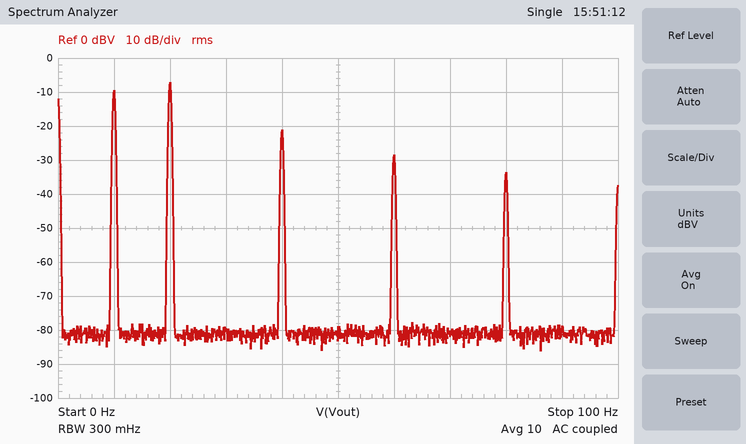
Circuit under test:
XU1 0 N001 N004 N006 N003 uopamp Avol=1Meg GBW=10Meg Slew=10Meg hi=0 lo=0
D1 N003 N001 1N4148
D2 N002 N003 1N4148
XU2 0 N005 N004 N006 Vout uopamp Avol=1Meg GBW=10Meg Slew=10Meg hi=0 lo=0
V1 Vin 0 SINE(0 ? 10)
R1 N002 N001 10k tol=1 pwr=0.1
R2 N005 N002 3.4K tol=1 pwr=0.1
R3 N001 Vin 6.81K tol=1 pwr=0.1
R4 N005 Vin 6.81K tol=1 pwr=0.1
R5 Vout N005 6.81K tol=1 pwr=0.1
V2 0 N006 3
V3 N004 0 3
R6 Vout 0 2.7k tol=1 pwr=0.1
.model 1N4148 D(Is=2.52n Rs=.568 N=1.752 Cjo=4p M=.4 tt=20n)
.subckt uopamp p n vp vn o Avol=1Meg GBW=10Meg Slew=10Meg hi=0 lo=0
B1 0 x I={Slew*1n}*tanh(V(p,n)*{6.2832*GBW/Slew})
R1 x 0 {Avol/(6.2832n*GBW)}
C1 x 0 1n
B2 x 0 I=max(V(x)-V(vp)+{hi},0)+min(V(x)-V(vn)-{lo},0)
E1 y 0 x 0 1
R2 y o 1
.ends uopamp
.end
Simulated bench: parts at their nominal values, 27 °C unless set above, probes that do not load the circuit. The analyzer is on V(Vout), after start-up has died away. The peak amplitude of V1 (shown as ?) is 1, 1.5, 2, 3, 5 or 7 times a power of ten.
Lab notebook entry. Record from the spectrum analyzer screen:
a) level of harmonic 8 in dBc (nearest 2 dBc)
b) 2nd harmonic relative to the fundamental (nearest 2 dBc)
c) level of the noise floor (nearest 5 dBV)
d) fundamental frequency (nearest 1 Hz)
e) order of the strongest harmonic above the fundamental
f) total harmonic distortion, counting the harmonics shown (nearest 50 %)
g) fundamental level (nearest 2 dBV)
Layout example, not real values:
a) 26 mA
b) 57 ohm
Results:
a) -24 dBc
b) 2 dBc
c) -80 dBV
d) 10 Hz
e) 2
f) 150 %
g) -10 dBV
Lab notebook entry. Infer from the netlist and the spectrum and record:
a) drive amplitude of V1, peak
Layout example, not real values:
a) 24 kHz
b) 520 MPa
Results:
a) 1 V
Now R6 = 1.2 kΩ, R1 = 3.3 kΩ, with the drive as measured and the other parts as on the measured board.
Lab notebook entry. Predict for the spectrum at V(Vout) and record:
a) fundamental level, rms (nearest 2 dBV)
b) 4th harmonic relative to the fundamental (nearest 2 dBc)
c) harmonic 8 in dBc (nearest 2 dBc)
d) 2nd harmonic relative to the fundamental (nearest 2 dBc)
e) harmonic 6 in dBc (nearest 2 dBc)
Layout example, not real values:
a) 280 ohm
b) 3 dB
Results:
a) -8 dBV
b) -22 dBc
c) -34 dBc
d) -8 dBc
e) -30 dBc
